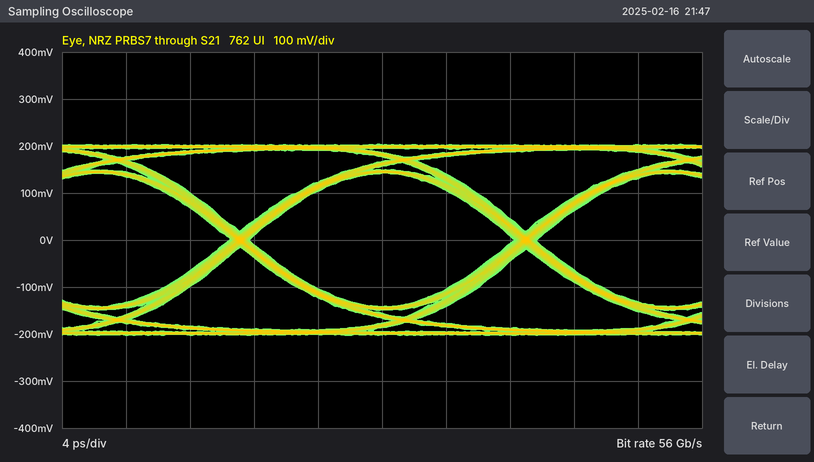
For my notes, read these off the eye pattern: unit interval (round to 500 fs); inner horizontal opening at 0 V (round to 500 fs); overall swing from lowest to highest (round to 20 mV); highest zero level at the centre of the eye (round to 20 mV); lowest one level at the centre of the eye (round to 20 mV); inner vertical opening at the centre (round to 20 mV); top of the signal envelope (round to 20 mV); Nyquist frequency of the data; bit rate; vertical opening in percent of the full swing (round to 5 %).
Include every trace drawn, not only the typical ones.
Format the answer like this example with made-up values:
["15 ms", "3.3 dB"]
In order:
["18.0 ps", "16.5 ps", "400 mV", "-140 mV", "140 mV", "280 mV", "200 mV", "28 GHz", "56 Gb/s", "70 %"]
